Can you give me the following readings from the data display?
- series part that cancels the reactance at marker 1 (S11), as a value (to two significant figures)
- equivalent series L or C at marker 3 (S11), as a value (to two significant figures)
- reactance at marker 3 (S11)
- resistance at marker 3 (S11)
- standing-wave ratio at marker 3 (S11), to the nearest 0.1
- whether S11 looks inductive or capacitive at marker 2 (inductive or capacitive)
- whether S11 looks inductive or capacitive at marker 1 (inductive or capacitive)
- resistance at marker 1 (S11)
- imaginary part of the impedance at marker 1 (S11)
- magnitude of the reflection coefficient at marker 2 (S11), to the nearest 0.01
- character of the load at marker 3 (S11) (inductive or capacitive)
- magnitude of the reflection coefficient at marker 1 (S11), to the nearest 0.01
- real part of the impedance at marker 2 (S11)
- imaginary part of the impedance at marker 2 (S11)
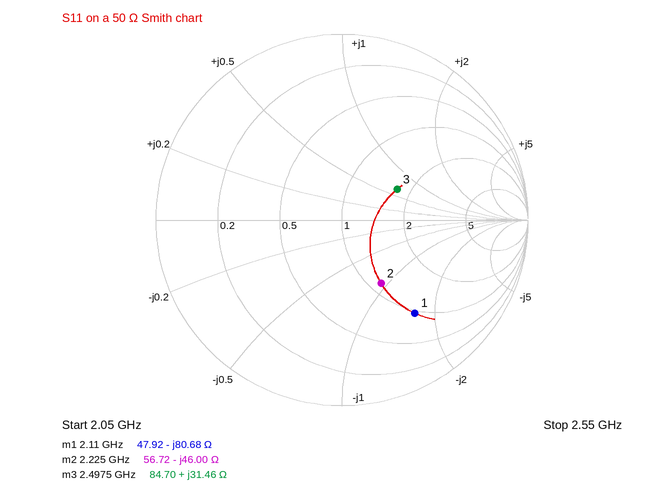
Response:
6.1 nH
2.0 nH
+31.46 Ω
84.70 Ω
2.0
capacitive
capacitive
47.92 Ω
-80.68 Ω
0.40
inductive
0.64
56.72 Ω
-46.00 Ω
